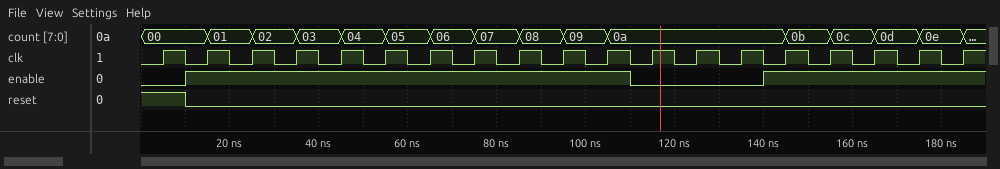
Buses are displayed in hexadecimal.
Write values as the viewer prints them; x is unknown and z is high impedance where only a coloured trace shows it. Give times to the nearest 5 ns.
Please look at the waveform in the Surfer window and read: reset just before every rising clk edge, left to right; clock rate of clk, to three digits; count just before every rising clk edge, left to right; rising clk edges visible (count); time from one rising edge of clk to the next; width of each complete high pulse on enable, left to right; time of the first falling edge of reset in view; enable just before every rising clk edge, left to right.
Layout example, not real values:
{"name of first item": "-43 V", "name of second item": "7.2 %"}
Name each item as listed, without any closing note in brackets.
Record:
{"reset just before every rising clk edge, left to right": "1 0 0 0 0 0 0 0 0 0 0 0 0 0 0 0 0 0 0", "clock rate of clk, to three digits": "100 MHz", "count just before every rising clk edge, left to right": "00, 00, 01, 02, 03, 04, 05, 06, 07, 08, 09, 0a, 0a, 0a, 0a, 0b, 0c, 0d, 0e", "rising clk edges visible": "19", "time from one rising edge of clk to the next": "10 ns", "width of each complete high pulse on enable, left to right": "100 ns", "time of the first falling edge of reset in view": "10 ns", "enable just before every rising clk edge, left to right": "0 1 1 1 1 1 1 1 1 1 1 0 0 0 1 1 1 1 1"}
